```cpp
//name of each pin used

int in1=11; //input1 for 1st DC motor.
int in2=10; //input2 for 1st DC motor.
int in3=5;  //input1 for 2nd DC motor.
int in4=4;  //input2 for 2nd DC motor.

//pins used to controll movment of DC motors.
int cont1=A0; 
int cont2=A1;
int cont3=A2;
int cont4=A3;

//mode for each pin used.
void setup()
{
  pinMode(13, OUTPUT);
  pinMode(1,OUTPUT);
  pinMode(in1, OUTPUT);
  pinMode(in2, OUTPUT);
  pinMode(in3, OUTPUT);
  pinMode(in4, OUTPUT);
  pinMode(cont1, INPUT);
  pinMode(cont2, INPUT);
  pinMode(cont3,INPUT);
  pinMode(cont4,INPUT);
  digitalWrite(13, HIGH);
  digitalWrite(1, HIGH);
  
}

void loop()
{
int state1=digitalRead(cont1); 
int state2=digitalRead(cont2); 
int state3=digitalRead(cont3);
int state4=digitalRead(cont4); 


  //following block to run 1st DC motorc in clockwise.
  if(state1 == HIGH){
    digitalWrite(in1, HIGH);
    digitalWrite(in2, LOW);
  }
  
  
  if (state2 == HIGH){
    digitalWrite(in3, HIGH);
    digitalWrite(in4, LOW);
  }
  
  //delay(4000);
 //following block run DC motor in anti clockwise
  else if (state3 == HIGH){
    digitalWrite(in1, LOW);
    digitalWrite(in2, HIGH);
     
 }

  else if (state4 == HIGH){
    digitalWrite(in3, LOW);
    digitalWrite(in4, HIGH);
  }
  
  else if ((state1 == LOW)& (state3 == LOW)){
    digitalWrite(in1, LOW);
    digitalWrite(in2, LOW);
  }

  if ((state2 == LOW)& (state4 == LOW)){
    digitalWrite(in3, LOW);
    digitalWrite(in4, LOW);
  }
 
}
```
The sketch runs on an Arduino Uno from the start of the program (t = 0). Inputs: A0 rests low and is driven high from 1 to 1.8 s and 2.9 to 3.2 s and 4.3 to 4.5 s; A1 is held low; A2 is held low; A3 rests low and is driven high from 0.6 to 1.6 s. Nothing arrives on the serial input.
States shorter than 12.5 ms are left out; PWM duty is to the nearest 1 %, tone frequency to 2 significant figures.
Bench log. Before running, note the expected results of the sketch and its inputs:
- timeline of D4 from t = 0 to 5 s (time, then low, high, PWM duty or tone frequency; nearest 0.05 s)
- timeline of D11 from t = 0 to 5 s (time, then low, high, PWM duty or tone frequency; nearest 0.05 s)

0 s low; 0.6 s high; 1.6 s low
0 s low; 1 s high; 1.8 s low; 2.9 s high; 3.2 s low; 4.3 s high; 4.5 s low
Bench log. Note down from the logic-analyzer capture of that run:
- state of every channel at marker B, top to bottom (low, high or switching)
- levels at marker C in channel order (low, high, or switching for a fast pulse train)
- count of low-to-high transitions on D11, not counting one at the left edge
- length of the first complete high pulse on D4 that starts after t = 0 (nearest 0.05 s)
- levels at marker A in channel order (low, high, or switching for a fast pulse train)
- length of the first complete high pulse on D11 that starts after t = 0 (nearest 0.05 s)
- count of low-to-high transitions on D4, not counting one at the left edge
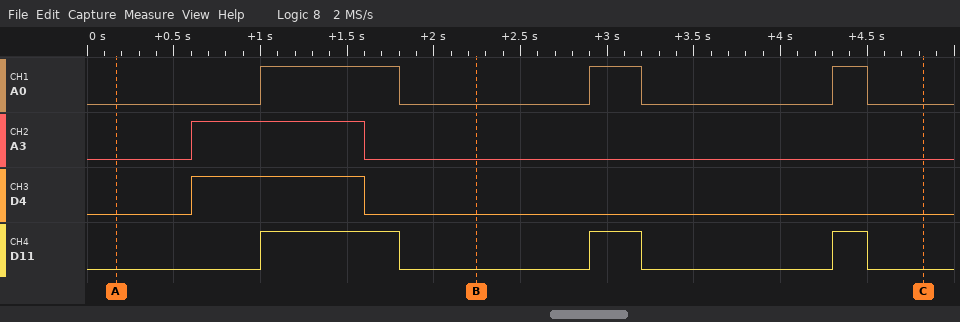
A0 low, A3 low, D4 low, D11 low
A0 low, A3 low, D4 low, D11 low
3
1.00 s
A0 low, A3 low, D4 low, D11 low
0.80 s
1
